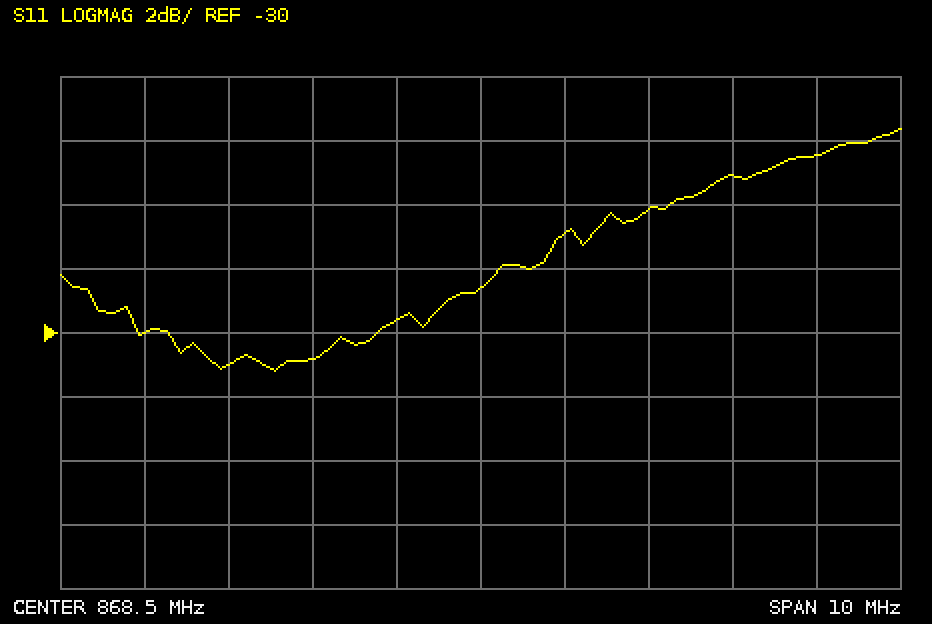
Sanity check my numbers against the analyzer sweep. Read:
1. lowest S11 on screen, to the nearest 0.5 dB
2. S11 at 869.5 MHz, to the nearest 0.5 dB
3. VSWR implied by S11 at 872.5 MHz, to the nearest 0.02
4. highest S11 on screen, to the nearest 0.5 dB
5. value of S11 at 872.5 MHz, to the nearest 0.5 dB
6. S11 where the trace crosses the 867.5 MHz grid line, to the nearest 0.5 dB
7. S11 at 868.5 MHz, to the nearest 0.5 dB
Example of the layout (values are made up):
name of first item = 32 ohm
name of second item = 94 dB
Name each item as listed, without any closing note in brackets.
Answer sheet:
lowest S11 on screen, to the nearest 0.5 dB = -31.0 dB
S11 at 869.5 MHz, to the nearest 0.5 dB = -27.0 dB
VSWR implied by S11 at 872.5 MHz, to the nearest 0.02 = 1.12
highest S11 on screen, to the nearest 0.5 dB = -23.5 dB
value of S11 at 872.5 MHz, to the nearest 0.5 dB = -24.5 dB
S11 where the trace crosses the 867.5 MHz grid line, to the nearest 0.5 dB = -29.5 dB
S11 at 868.5 MHz, to the nearest 0.5 dB = -28.5 dB
